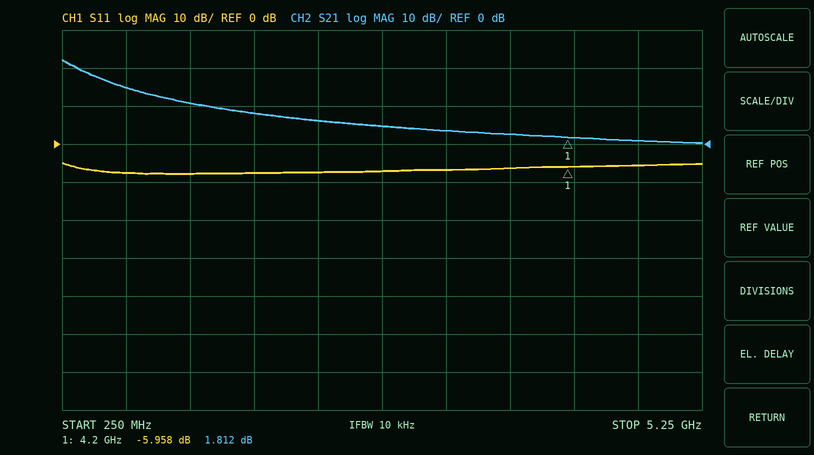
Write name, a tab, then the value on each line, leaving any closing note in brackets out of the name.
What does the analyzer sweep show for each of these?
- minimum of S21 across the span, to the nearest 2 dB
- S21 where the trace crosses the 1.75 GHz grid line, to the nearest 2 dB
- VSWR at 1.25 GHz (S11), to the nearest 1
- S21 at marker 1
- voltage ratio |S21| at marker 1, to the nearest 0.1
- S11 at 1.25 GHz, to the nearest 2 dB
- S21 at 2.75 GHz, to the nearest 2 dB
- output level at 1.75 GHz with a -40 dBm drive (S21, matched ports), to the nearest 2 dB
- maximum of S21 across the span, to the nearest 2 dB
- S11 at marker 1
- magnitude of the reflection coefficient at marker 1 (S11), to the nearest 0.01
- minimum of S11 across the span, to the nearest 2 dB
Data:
minimum of S21 across the span, to the nearest 2 dB	0 dB
S21 where the trace crosses the 1.75 GHz grid line, to the nearest 2 dB	8 dB
VSWR at 1.25 GHz (S11), to the nearest 1	2
S21 at marker 1	1.812 dB
voltage ratio |S21| at marker 1, to the nearest 0.1	1.2
S11 at 1.25 GHz, to the nearest 2 dB	-8 dB
S21 at 2.75 GHz, to the nearest 2 dB	4 dB
output level at 1.75 GHz with a -40 dBm drive (S21, matched ports), to the nearest 2 dB	-32 dBm
maximum of S21 across the span, to the nearest 2 dB	22 dB
S11 at marker 1	-5.958 dB
magnitude of the reflection coefficient at marker 1 (S11), to the nearest 0.01	0.50
minimum of S11 across the span, to the nearest 2 dB	-8 dB
